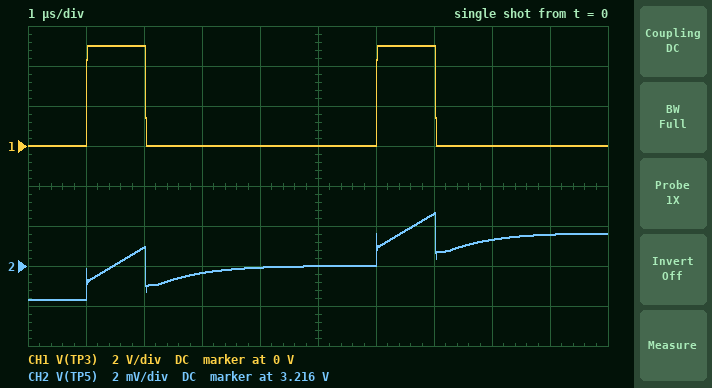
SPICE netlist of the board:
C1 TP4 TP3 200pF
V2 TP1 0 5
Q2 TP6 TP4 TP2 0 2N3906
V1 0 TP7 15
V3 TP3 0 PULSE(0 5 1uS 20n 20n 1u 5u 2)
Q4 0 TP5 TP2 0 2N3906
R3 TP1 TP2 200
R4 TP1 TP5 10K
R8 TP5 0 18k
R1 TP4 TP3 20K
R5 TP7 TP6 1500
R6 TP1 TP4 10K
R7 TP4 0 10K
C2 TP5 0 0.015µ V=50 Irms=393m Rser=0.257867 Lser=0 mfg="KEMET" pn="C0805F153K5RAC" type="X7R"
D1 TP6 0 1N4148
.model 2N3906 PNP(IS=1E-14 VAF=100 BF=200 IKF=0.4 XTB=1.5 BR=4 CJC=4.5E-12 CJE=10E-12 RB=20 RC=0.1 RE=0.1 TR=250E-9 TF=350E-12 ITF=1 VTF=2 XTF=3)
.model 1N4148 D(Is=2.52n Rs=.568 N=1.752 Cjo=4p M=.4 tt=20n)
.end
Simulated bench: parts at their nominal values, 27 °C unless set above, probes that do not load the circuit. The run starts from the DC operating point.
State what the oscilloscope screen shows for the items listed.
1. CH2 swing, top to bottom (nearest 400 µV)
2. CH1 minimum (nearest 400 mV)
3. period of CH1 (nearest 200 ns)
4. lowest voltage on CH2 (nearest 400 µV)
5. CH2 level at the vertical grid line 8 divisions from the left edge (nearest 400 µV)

4.4 mV
0 V
5.0 µs
3.2144 V
3.2172 V
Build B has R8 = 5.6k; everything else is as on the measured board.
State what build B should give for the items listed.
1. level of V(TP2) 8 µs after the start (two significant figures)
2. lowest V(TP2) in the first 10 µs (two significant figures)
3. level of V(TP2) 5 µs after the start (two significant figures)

2.2 V
680 mV
2.7 V
